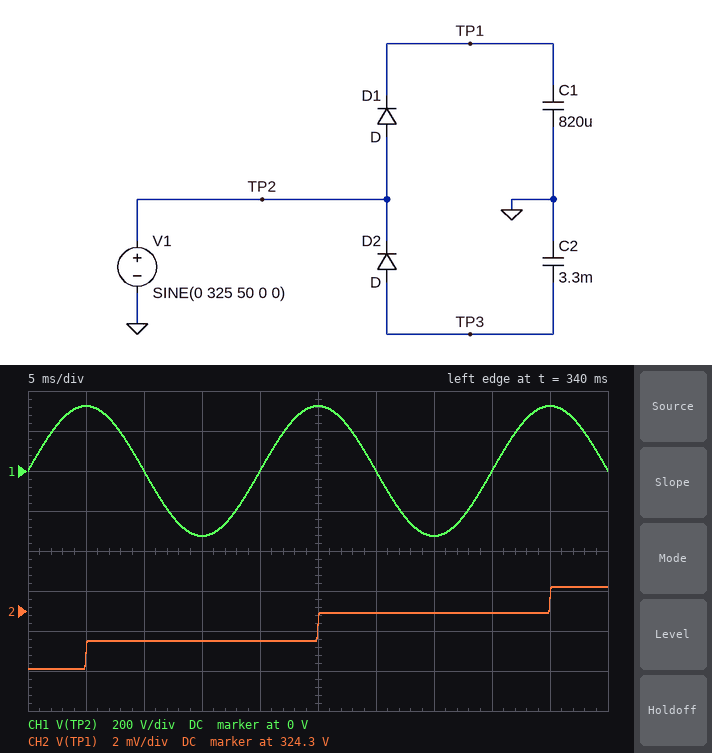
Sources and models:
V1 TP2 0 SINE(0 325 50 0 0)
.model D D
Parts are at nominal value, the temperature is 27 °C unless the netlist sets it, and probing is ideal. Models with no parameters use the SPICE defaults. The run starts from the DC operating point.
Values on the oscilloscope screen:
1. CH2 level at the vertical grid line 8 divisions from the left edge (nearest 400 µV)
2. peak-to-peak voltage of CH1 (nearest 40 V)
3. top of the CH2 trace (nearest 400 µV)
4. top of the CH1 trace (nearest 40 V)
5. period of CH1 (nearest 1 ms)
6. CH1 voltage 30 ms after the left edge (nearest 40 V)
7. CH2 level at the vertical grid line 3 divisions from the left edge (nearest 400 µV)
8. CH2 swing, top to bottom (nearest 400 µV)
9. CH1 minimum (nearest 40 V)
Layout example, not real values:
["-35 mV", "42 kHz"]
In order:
["324.2740 V", "640 V", "324.2752 V", "320 V", "20 ms", "0 V", "324.2724 V", "4.0 mV", "-320 V"]
